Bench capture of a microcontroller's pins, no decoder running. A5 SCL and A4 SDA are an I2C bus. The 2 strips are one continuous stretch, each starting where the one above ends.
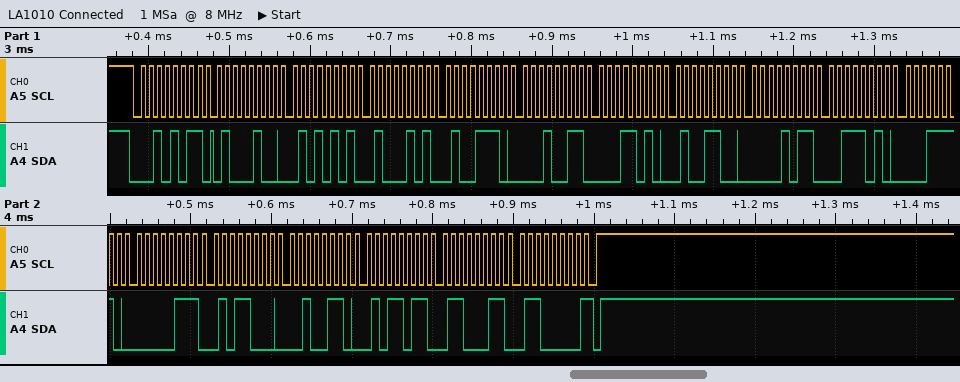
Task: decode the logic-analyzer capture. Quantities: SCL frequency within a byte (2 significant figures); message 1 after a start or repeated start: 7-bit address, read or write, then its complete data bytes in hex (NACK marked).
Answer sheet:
100 kHz
0x15 read: 44 55 45 4E 13 1A 4C 0B 3A 1E 07 58 26 5B 63 60 NACK
